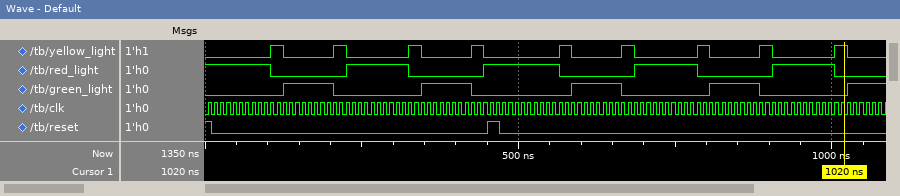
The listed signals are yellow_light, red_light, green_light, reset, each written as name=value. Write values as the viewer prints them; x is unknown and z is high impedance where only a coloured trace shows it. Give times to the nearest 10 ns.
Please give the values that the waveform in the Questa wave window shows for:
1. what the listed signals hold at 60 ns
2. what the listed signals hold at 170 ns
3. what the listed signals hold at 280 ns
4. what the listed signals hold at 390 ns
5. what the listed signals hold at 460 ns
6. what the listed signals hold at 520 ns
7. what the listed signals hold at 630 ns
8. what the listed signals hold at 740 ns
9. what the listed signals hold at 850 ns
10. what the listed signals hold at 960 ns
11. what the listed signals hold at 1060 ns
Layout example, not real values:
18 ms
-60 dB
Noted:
yellow_light=0, red_light=1, green_light=0, reset=0
yellow_light=0, red_light=0, green_light=1, reset=0
yellow_light=0, red_light=1, green_light=0, reset=0
yellow_light=0, red_light=0, green_light=1, reset=0
yellow_light=0, red_light=1, green_light=0, reset=1
yellow_light=0, red_light=1, green_light=0, reset=0
yellow_light=0, red_light=0, green_light=1, reset=0
yellow_light=0, red_light=1, green_light=0, reset=0
yellow_light=0, red_light=0, green_light=1, reset=0
yellow_light=0, red_light=1, green_light=0, reset=0
yellow_light=0, red_light=0, green_light=1, reset=0
